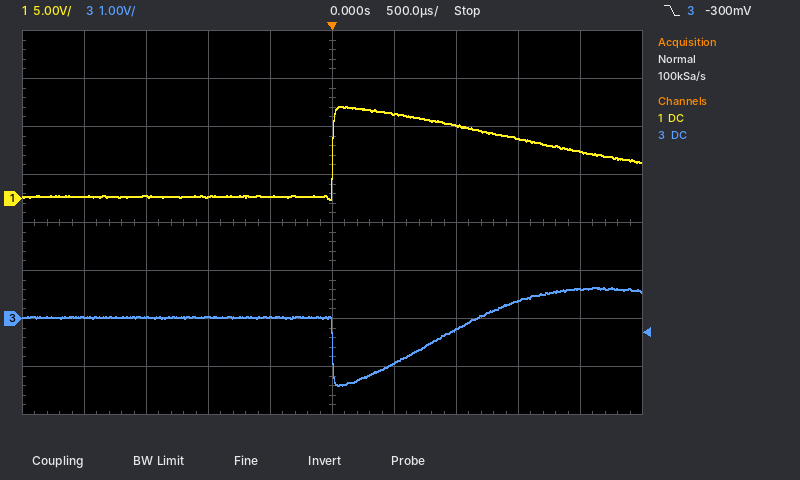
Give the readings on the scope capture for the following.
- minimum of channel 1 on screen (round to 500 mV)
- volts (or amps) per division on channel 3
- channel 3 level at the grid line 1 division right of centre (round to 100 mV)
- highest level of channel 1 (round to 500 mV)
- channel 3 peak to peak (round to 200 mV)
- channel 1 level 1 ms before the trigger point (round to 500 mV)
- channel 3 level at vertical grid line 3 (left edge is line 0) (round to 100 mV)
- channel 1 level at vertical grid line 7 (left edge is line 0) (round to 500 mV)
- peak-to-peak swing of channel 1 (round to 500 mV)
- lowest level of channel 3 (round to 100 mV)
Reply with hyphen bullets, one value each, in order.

- 0.0 V
- 1 V
- -900 mV
- 9.5 V
- 2.0 V
- 0.0 V
- 0.0 V
- 7.5 V
- 9.5 V
- -1.4 V
